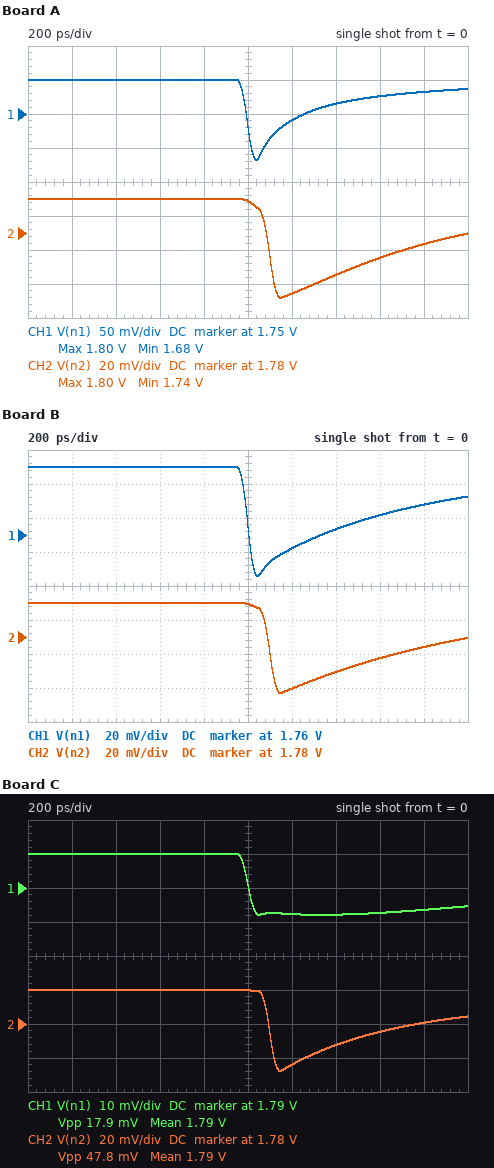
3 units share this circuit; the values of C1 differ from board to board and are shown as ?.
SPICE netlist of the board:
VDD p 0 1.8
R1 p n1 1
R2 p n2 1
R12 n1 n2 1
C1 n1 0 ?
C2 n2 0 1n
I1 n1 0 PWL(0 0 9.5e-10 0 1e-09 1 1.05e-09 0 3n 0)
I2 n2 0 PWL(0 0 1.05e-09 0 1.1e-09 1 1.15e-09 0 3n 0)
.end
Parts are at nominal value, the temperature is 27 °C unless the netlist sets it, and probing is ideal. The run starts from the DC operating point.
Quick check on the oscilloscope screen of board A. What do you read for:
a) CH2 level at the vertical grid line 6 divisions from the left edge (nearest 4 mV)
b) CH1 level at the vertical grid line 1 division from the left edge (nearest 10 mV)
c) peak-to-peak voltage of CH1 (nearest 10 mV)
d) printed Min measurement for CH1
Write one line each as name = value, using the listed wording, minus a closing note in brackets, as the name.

CH2 level at the vertical grid line 6 divisions from the left edge = 1.744 V
CH1 level at the vertical grid line 1 division from the left edge = 1.80 V
peak-to-peak voltage of CH1 = 120 mV
printed Min measurement for CH1 = 1.68 V
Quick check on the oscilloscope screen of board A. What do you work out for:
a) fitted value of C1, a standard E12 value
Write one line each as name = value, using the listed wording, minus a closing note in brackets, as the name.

fitted value of C1, a standard E12 value = 330 pF
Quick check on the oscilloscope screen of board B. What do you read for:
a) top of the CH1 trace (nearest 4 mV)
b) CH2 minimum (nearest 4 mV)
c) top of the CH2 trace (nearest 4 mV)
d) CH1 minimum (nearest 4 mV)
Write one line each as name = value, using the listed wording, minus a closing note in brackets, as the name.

top of the CH1 trace = 1.800 V
CH2 minimum = 1.748 V
top of the CH2 trace = 1.800 V
CH1 minimum = 1.736 V
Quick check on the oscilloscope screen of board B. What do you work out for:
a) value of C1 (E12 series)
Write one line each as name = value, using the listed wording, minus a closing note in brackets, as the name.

value of C1 = 680 pF
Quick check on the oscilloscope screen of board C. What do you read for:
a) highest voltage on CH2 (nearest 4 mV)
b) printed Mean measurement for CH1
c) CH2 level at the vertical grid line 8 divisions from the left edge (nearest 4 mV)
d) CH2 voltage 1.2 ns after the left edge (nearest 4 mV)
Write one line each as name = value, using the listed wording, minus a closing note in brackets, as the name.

highest voltage on CH2 = 1.800 V
printed Mean measurement for CH1 = 1.79 V
CH2 level at the vertical grid line 8 divisions from the left edge = 1.776 V
CH2 voltage 1.2 ns after the left edge = 1.756 V
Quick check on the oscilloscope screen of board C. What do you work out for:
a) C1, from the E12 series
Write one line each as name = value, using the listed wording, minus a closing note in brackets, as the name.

C1, from the E12 series = 2.7 nF
